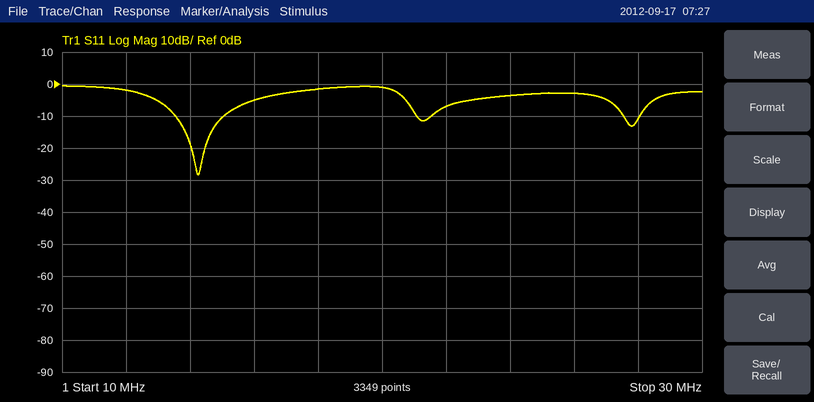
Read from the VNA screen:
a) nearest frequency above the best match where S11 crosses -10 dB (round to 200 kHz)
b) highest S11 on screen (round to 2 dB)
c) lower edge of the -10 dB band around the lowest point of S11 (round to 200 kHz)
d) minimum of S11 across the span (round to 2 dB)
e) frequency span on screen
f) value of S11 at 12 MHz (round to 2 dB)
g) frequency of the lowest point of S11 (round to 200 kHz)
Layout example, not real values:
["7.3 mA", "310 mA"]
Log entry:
["15.0 MHz", "0 dB", "13.6 MHz", "-28 dB", "20 MHz", "-2 dB", "14.2 MHz"]
